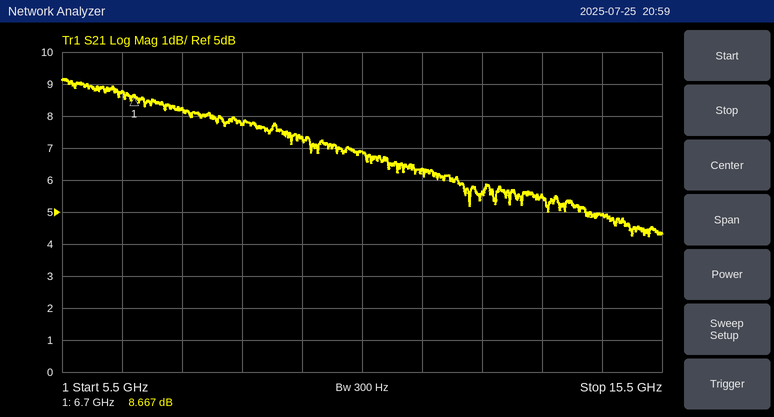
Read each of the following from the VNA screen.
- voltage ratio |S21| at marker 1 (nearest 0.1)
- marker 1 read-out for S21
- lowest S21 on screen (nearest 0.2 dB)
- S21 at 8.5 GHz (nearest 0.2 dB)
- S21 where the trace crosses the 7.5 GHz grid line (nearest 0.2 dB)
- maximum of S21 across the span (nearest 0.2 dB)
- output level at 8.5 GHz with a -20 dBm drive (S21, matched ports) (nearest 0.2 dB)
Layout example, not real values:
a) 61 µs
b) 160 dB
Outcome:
a) 2.7
b) 8.667 dB
c) 4.2 dB
d) 7.8 dB
e) 8.2 dB
f) 9.2 dB
g) -12.2 dBm
